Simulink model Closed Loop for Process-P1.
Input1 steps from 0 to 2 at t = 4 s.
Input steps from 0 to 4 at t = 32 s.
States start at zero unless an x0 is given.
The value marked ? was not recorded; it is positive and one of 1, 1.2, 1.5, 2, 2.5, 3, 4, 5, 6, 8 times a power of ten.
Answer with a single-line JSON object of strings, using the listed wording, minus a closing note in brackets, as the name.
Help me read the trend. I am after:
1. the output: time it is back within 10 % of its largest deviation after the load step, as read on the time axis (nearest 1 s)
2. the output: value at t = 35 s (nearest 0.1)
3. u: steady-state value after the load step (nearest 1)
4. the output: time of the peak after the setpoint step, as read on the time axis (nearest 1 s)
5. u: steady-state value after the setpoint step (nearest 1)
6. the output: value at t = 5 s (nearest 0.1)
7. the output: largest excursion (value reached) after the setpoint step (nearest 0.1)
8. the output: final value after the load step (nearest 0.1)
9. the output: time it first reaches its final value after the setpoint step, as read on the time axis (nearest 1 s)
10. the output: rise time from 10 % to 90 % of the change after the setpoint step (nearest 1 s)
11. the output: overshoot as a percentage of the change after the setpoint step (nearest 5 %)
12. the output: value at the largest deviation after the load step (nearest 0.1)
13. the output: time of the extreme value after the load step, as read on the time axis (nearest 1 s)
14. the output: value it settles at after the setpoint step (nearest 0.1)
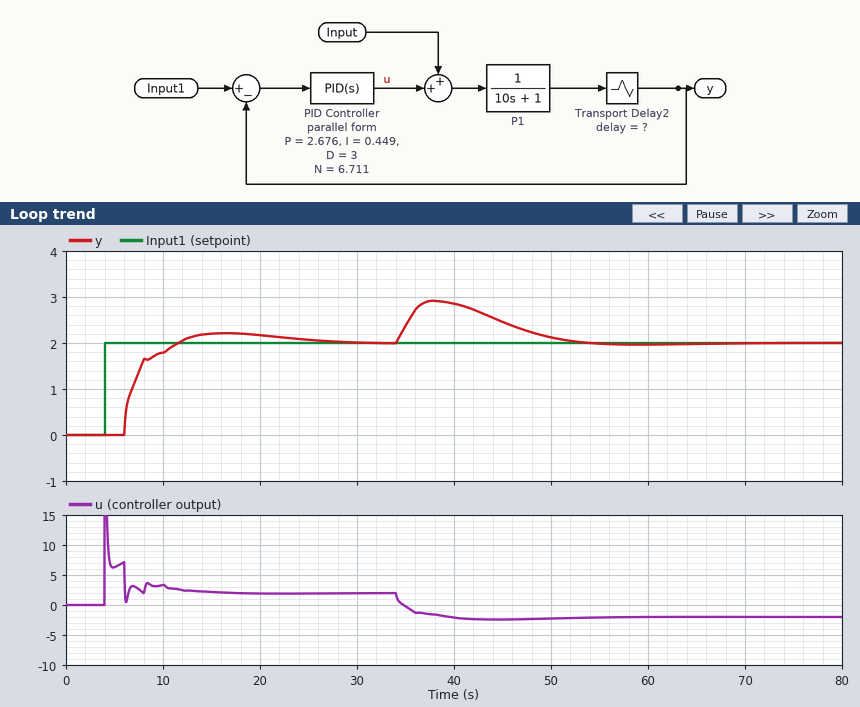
{"the output: time it is back within 10 % of its largest deviation after the load step, as read on the time axis": "51 s", "the output: value at t = 35 s": "2.4", "u: steady-state value after the load step": "-2", "the output: time of the peak after the setpoint step, as read on the time axis": "17 s", "u: steady-state value after the setpoint step": "2", "the output: value at t = 5 s": "0.0", "the output: largest excursion (value reached) after the setpoint step": "2.2", "the output: final value after the load step": "2.0", "the output: time it first reaches its final value after the setpoint step, as read on the time axis": "12 s", "the output: rise time from 10 % to 90 % of the change after the setpoint step": "4 s", "the output: overshoot as a percentage of the change after the setpoint step": "10 %", "the output: value at the largest deviation after the load step": "2.9", "the output: time of the extreme value after the load step, as read on the time axis": "38 s", "the output: value it settles at after the setpoint step": "2.0"}
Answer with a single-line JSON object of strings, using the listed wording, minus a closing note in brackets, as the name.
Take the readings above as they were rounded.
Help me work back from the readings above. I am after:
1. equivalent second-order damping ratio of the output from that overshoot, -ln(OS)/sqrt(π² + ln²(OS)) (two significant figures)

{"equivalent second-order damping ratio of the output from that overshoot, -ln(OS)/sqrt(π² + ln²(OS))": "0.59"}
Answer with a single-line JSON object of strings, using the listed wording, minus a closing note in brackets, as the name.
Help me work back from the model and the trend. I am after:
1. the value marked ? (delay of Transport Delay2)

{"the value marked ?": "2"}
